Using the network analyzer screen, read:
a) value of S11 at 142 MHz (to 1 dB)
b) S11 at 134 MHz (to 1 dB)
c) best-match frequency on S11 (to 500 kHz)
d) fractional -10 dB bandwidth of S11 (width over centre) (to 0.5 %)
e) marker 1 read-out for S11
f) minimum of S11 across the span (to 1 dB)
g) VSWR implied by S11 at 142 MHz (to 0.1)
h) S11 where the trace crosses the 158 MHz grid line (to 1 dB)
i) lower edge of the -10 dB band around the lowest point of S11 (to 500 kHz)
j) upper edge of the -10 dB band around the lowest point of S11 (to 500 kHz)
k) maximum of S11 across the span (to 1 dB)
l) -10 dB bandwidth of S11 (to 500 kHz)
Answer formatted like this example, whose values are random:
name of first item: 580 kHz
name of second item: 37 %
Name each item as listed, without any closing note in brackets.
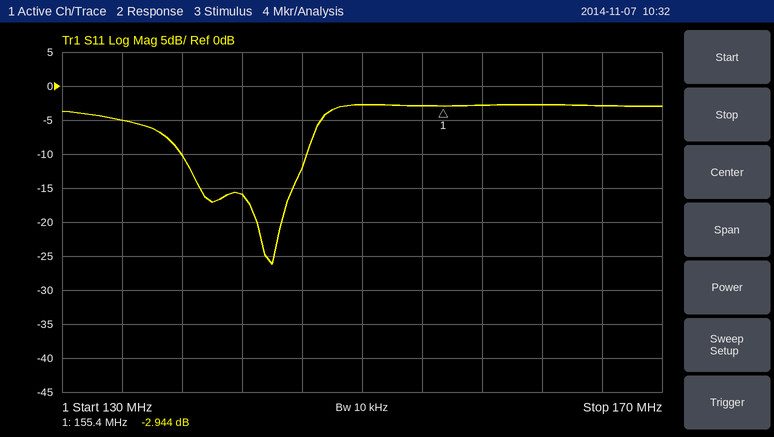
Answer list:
value of S11 at 142 MHz: -16 dB
S11 at 134 MHz: -5 dB
best-match frequency on S11: 144.0 MHz
fractional -10 dB bandwidth of S11 (width over centre): 6.0 %
marker 1 read-out for S11: -2.944 dB
minimum of S11 across the span: -26 dB
VSWR implied by S11 at 142 MHz: 1.4
S11 where the trace crosses the 158 MHz grid line: -3 dB
lower edge of the -10 dB band around the lowest point of S11: 138.0 MHz
upper edge of the -10 dB band around the lowest point of S11: 146.5 MHz
maximum of S11 across the span: -3 dB
-10 dB bandwidth of S11: 8.5 MHz
